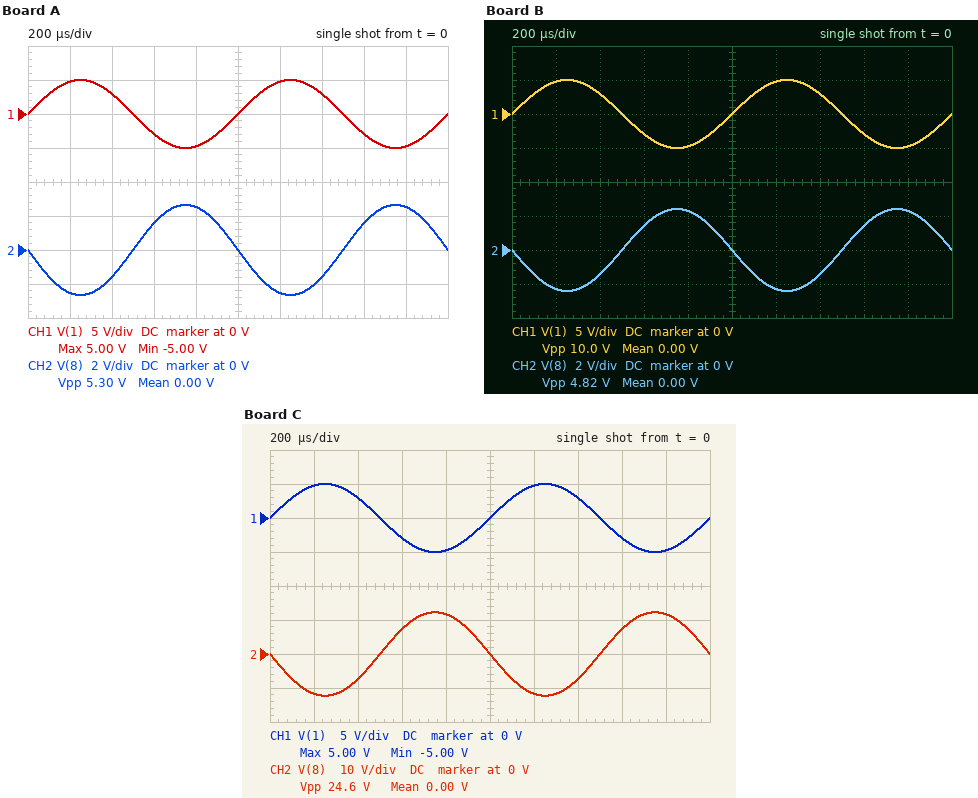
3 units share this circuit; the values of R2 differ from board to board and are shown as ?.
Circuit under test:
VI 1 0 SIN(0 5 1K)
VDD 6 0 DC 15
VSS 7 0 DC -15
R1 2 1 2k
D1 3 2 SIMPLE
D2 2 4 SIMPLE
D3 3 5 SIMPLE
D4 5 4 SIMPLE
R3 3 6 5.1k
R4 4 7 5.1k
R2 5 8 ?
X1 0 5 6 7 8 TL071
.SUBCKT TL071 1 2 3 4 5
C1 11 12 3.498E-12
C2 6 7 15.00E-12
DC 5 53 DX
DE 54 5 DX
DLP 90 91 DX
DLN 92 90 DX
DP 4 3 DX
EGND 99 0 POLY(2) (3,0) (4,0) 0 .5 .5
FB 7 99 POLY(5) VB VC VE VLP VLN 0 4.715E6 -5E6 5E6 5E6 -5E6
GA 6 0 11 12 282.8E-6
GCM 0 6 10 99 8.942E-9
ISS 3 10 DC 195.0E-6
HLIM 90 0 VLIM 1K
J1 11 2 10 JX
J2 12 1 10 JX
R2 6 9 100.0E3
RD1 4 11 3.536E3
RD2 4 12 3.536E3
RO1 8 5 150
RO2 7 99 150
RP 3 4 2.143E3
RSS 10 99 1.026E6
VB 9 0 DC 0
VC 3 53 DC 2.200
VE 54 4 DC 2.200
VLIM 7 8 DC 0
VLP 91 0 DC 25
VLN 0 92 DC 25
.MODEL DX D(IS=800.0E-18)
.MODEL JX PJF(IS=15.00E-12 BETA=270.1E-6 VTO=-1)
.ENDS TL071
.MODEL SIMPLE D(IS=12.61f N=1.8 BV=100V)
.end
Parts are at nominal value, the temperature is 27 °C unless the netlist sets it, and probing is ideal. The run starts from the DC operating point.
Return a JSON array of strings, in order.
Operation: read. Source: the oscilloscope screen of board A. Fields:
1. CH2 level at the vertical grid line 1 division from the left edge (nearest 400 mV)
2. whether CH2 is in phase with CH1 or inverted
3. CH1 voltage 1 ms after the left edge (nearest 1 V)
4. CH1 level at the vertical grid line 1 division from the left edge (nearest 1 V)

["-2.4 V", "inverted", "0 V", "5 V"]
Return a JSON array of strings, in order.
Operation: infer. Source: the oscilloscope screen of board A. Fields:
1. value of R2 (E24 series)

["1.1 kΩ"]
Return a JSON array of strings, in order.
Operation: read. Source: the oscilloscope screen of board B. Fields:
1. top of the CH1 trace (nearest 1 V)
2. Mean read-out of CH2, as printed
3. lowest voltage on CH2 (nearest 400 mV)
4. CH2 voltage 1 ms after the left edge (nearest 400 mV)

["5 V", "0.00 V", "-2.4 V", "0 V"]
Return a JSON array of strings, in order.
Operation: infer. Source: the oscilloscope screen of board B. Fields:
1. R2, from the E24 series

["1 kΩ"]
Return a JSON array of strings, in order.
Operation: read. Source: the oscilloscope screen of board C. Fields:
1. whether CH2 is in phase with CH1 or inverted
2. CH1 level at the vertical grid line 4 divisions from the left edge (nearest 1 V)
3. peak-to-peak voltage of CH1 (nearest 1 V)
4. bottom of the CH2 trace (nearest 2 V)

["inverted", "-5 V", "10 V", "-12 V"]
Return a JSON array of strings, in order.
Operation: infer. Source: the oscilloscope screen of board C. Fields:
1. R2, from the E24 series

["5.1 kΩ"]
